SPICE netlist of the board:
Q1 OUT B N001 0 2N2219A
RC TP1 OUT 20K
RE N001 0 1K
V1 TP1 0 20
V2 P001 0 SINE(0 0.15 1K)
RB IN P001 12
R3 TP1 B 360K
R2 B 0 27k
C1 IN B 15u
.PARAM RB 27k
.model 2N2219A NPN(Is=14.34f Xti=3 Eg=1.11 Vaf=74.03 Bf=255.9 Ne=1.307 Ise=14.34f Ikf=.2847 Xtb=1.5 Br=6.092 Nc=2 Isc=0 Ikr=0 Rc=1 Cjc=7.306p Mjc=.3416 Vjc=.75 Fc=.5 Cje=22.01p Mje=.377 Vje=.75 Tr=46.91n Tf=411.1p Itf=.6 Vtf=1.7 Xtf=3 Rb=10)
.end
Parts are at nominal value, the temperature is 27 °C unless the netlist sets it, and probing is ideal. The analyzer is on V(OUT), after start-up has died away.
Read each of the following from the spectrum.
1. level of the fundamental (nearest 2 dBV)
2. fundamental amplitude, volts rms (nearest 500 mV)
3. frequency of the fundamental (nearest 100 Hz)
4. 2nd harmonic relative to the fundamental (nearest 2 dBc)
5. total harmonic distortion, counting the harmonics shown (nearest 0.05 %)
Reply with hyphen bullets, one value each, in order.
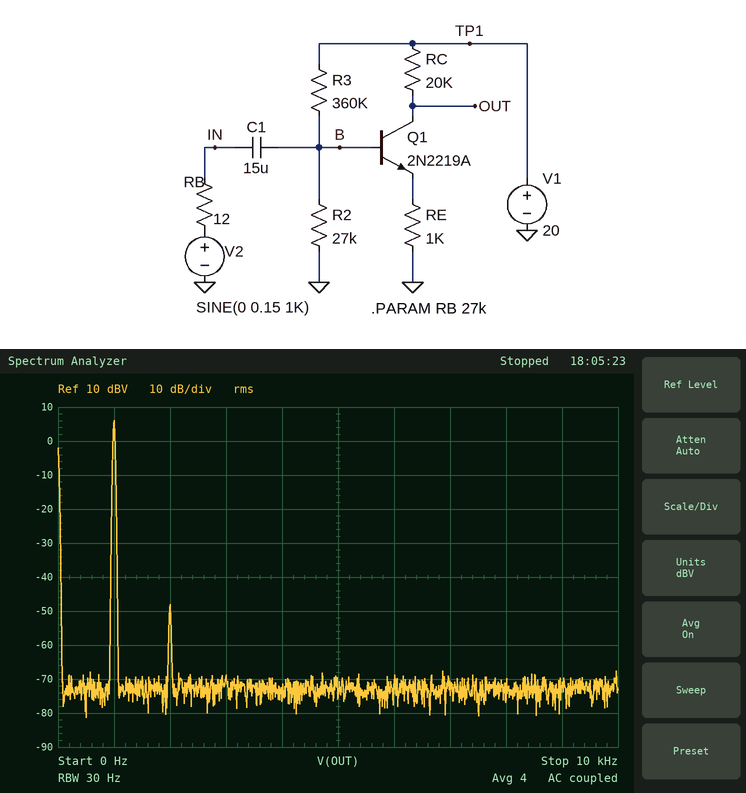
- 6 dBV
- 2.0 V
- 1.0 kHz
- -54 dBc
- 0.20 %
